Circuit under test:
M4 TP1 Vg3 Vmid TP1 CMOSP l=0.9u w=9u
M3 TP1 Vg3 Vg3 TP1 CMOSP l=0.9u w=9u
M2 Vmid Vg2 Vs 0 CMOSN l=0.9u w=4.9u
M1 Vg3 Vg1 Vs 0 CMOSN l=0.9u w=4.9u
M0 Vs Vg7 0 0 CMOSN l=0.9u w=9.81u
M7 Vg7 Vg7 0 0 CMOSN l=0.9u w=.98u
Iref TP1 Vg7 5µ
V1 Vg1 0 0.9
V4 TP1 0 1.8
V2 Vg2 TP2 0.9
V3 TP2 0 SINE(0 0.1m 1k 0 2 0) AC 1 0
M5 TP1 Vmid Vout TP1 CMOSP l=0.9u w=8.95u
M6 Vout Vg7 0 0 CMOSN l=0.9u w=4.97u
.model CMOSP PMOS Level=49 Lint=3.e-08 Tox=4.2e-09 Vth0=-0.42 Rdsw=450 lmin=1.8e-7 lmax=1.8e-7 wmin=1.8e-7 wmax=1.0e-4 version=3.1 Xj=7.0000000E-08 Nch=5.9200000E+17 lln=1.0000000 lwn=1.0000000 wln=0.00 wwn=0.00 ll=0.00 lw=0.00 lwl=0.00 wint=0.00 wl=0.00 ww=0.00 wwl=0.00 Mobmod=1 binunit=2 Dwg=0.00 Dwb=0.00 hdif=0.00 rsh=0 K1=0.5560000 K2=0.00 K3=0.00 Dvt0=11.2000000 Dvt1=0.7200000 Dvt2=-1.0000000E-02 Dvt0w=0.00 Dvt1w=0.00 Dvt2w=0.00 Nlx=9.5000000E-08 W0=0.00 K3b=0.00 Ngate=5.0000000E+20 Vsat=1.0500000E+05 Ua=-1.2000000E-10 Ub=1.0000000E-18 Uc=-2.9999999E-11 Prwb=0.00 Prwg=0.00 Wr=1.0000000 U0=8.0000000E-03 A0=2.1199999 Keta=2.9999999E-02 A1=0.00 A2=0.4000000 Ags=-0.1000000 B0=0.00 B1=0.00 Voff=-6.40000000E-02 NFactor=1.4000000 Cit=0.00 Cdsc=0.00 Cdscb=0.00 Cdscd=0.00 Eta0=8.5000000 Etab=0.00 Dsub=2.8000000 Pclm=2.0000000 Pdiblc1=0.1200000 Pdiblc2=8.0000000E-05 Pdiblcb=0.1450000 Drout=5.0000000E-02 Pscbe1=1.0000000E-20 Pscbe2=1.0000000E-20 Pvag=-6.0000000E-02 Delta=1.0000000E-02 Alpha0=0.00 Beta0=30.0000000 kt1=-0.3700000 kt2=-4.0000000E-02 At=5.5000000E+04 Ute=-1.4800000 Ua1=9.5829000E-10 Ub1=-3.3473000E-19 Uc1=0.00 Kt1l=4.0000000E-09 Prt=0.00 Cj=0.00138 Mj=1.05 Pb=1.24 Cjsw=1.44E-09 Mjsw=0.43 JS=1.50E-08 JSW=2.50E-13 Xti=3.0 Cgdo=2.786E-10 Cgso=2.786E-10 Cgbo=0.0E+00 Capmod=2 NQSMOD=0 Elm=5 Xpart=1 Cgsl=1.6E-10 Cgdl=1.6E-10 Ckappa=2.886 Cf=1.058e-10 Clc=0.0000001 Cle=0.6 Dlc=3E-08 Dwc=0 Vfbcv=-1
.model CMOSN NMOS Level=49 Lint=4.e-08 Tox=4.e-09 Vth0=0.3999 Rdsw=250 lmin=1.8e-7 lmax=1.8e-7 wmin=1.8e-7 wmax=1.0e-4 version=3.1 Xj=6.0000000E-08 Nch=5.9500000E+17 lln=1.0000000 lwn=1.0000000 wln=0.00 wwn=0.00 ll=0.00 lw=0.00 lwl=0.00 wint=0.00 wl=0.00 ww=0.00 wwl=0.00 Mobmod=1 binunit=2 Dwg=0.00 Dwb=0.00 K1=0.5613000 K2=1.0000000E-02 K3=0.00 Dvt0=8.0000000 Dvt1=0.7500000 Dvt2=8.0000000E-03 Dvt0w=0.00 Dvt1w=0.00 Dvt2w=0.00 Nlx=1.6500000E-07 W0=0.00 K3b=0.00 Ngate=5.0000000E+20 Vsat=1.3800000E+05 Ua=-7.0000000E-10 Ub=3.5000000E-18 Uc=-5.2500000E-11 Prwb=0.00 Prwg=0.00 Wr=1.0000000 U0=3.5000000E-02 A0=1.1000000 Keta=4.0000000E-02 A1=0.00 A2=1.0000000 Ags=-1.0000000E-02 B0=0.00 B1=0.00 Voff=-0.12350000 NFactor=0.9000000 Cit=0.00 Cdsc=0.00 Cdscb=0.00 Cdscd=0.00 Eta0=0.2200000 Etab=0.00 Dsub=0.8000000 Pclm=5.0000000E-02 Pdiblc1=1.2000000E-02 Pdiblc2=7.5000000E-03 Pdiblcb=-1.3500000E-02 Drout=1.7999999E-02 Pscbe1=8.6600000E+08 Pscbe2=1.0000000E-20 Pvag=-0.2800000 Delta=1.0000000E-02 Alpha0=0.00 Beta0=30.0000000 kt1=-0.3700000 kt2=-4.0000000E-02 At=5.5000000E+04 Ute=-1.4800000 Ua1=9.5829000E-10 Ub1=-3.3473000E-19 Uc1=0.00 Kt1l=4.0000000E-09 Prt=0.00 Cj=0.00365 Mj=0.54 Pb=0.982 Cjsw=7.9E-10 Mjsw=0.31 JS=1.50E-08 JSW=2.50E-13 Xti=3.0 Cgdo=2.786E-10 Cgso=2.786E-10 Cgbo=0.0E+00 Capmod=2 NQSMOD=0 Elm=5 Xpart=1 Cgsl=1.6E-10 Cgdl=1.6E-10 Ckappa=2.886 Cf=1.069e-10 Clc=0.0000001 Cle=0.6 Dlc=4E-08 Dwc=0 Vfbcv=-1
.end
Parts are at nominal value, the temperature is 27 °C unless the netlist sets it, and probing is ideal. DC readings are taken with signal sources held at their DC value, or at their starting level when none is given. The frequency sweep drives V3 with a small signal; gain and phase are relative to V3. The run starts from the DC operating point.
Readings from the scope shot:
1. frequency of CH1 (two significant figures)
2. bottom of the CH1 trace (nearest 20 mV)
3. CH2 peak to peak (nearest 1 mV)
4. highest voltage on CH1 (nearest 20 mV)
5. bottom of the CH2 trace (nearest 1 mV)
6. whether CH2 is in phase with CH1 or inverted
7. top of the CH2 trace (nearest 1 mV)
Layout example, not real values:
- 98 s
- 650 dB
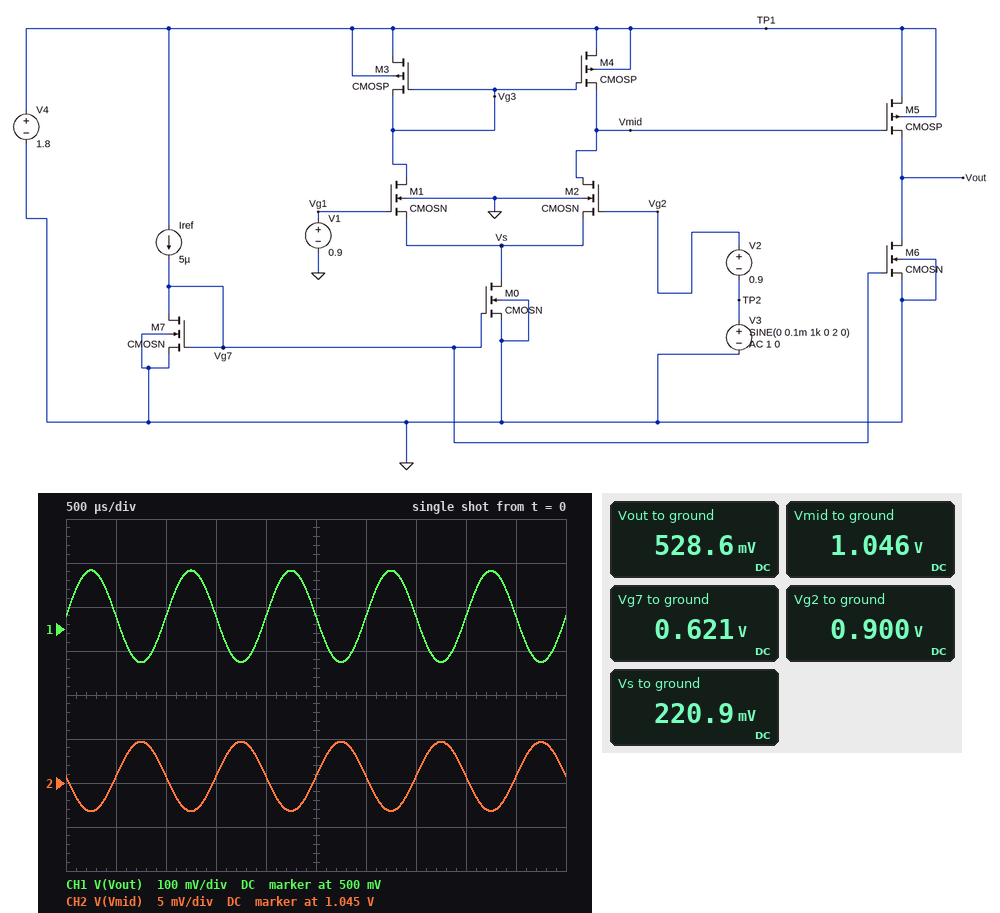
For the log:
- 1.0 kHz
- 420 mV
- 8 mV
- 640 mV
- 1.042 V
- inverted
- 1.050 V
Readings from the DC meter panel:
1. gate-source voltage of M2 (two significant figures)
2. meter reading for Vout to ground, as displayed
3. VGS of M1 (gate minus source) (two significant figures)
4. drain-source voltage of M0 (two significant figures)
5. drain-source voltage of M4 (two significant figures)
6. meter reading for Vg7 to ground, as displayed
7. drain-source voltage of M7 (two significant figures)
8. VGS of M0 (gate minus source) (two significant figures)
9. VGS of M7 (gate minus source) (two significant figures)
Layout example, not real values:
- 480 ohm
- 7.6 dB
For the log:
- 680 mV
- 528.6 mV
- 680 mV
- 220 mV
- 750 mV
- 0.621 V
- 620 mV
- 620 mV
- 620 mV
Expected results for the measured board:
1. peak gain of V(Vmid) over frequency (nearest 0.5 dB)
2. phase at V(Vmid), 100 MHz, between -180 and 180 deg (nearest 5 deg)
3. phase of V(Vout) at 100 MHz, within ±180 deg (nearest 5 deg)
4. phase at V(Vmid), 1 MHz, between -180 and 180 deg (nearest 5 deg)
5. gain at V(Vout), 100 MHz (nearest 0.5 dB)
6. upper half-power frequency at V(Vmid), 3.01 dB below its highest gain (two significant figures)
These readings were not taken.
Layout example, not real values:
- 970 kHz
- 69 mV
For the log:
- 32.0 dB
- 85 deg
- -160 deg
- 165 deg
- 27.0 dB
- 4.0 MHz
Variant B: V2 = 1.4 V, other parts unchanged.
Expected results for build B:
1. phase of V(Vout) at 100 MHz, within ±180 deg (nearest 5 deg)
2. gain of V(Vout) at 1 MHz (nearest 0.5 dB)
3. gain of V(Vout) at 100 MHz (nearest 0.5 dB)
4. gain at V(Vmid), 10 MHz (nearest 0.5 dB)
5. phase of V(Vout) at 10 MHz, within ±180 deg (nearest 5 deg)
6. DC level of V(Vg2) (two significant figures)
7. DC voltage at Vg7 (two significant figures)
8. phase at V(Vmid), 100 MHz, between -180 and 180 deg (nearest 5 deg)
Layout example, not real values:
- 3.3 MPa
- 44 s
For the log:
- -100 deg
- -57.5 dB
- -47.0 dB
- -29.0 dB
- -15 deg
- 1.4 V
- 620 mV
- 120 deg
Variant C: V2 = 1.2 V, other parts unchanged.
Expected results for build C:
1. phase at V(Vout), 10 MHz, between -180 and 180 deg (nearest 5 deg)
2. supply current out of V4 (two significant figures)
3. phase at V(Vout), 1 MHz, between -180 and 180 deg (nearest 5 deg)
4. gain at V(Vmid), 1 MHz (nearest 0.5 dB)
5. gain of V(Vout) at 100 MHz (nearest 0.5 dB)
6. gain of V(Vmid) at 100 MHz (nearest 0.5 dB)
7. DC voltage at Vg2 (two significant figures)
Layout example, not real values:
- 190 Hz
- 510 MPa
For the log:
- -10 deg
- 81 µA
- 0 deg
- -21.5 dB
- -43.0 dB
- -19.0 dB
- 1.2 V
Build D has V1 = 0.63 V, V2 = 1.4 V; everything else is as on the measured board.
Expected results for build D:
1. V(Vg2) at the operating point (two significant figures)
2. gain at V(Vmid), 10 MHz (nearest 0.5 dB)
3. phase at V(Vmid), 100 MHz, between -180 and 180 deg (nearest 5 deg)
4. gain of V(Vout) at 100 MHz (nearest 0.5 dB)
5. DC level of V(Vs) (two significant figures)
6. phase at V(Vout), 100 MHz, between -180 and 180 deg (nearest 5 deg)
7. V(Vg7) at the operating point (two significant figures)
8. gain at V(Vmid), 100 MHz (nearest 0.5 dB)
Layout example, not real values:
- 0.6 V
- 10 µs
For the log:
- 1.4 V
- -39.5 dB
- 100 deg
- -49.5 dB
- 61 mV
- -100 deg
- 620 mV
- -27.0 dB
